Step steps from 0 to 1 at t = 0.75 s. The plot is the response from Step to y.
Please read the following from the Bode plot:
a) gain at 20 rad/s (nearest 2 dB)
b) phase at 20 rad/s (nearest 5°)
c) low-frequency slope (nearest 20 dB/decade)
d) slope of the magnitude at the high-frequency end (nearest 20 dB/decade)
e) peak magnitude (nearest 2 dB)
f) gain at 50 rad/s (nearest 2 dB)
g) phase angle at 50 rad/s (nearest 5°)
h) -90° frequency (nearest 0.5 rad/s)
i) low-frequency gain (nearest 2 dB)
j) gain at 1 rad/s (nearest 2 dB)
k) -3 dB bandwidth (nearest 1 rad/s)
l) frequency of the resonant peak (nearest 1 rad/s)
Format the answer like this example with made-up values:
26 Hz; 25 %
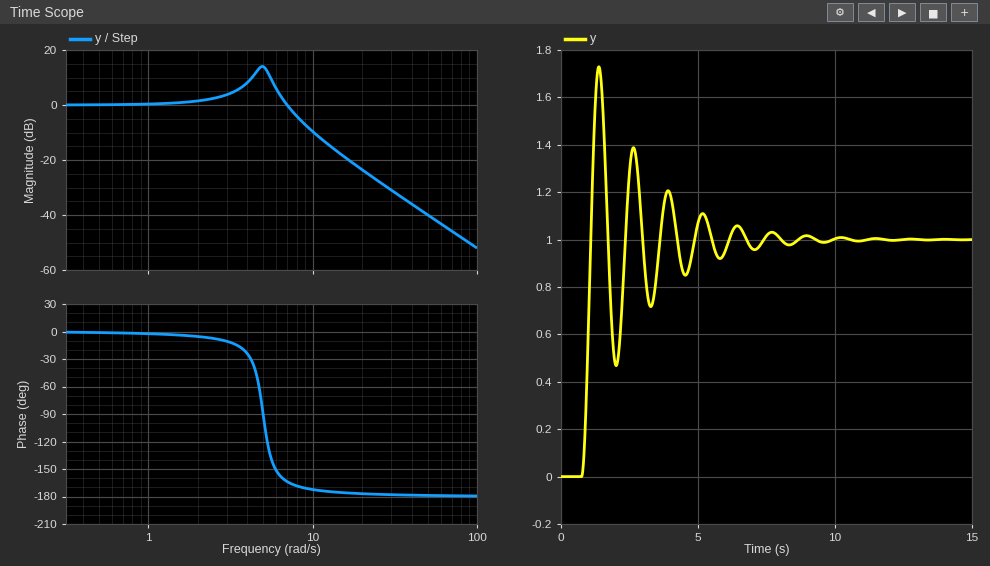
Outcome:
-24 dB; -175°; 0 dB/decade; -40 dB/decade; 14 dB; -40 dB; -180°; 5.0 rad/s; 0 dB; 0 dB; 8 rad/s; 5 rad/s
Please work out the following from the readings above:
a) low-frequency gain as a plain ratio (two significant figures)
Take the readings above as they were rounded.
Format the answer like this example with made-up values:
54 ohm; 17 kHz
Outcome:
1.0
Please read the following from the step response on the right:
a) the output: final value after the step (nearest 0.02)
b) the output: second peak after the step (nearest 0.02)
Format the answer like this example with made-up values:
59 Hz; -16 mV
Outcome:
1.00; 1.38
